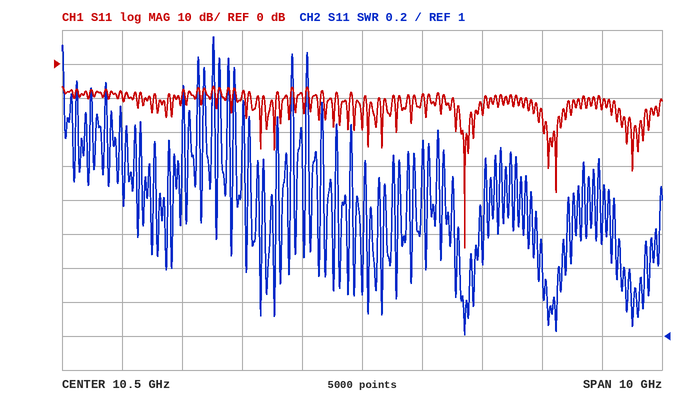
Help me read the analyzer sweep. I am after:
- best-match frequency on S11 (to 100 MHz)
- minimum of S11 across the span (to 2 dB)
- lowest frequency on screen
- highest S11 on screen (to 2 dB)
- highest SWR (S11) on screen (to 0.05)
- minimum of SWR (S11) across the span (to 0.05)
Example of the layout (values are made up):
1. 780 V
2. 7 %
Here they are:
1. 12.2 GHz
2. -54 dB
3. 5.5 GHz
4. -6 dB
5. 2.75
6. 1.00
